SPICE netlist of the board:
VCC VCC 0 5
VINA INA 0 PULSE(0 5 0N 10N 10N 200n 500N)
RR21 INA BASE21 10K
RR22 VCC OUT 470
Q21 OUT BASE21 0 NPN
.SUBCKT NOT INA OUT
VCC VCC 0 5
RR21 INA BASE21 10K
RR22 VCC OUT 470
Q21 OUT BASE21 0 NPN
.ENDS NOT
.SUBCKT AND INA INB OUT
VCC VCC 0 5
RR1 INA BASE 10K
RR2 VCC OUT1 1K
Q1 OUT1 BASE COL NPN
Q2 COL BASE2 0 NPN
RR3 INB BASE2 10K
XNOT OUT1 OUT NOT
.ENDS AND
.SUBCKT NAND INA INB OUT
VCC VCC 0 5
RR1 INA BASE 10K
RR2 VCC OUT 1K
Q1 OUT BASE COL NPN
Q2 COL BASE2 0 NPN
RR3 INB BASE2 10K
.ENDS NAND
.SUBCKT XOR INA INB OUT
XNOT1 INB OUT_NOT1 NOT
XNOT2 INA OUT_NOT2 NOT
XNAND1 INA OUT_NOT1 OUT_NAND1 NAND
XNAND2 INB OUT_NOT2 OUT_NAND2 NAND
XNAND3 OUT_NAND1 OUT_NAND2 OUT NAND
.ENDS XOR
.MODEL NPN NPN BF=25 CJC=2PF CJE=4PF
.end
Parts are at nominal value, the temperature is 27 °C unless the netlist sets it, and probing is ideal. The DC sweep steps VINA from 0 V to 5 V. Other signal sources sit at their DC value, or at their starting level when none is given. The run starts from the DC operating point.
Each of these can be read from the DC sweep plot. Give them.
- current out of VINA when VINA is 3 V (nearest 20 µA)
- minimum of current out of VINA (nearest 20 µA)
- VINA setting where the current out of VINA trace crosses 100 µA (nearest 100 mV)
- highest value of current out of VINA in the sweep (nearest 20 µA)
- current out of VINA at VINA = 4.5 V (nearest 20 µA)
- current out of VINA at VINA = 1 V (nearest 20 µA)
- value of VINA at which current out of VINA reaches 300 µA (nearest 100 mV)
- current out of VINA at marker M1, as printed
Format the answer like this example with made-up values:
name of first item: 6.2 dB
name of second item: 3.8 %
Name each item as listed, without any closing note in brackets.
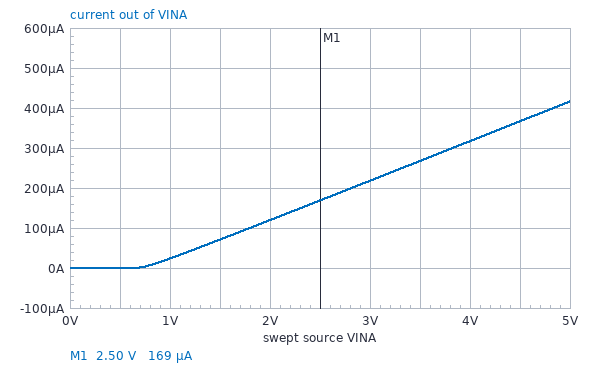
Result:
current out of VINA when VINA is 3 V: 220 µA
minimum of current out of VINA: 0 A
VINA setting where the current out of VINA trace crosses 100 µA: 1.8 V
highest value of current out of VINA in the sweep: 420 µA
current out of VINA at VINA = 4.5 V: 360 µA
current out of VINA at VINA = 1 V: 20 µA
value of VINA at which current out of VINA reaches 300 µA: 3.8 V
current out of VINA at marker M1, as printed: 169 µA
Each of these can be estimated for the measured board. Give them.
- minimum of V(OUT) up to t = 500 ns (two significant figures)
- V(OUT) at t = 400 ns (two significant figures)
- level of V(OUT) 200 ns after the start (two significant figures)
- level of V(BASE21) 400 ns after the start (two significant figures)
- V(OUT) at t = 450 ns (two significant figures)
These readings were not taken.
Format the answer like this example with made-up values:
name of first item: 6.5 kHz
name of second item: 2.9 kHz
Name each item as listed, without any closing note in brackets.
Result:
minimum of V(OUT) up to t = 500 ns: 190 mV
V(OUT) at t = 400 ns: 5.0 V
level of V(OUT) 200 ns after the start: 190 mV
level of V(BASE21) 400 ns after the start: 55 mV
V(OUT) at t = 450 ns: 5.0 V
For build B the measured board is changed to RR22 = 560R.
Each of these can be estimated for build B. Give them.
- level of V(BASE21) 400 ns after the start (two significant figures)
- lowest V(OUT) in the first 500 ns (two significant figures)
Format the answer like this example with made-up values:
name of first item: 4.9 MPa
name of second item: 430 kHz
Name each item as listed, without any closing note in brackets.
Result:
level of V(BASE21) 400 ns after the start: 59 mV
lowest V(OUT) in the first 500 ns: 130 mV
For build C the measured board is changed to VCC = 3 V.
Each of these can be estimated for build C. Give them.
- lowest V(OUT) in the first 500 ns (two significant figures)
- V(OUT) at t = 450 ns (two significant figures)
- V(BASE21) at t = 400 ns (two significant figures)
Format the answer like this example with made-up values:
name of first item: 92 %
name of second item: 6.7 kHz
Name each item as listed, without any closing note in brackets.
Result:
lowest V(OUT) in the first 500 ns: 96 mV
V(OUT) at t = 450 ns: 3.0 V
V(BASE21) at t = 400 ns: 59 mV
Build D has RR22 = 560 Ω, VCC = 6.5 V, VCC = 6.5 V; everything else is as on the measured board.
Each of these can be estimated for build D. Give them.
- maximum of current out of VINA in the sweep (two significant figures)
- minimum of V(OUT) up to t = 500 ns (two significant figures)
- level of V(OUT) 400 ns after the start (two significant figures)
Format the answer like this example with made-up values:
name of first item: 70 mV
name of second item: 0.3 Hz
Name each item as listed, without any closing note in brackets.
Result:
maximum of current out of VINA in the sweep: 420 µA
minimum of V(OUT) up to t = 500 ns: 670 mV
level of V(OUT) 400 ns after the start: 6.5 V
